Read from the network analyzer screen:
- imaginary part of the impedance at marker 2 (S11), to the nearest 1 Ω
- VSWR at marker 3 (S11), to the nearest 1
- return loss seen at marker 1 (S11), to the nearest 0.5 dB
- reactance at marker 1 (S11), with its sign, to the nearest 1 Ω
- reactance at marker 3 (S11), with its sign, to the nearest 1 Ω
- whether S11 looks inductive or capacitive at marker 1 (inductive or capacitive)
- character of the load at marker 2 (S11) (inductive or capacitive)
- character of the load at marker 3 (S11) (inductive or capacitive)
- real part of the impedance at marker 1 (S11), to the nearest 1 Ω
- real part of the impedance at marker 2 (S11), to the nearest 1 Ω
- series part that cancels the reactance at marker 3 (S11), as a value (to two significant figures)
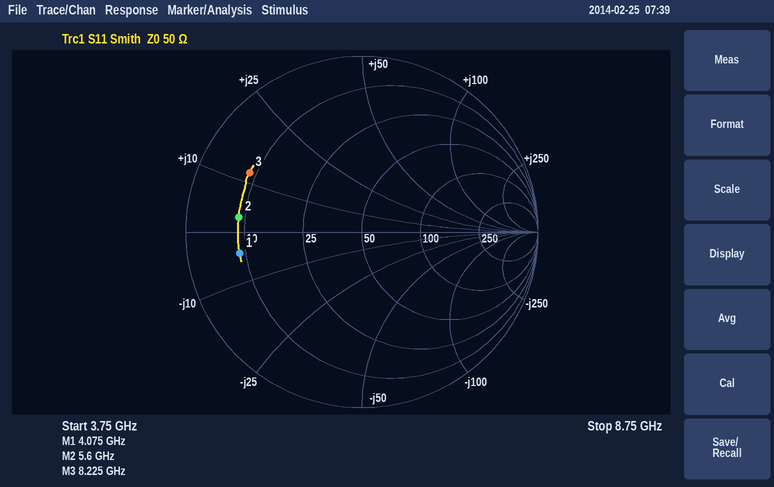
+3 Ω
6
3.0 dB
-4 Ω
+12 Ω
capacitive
inductive
inductive
9 Ω
9 Ω
1.6 pF
